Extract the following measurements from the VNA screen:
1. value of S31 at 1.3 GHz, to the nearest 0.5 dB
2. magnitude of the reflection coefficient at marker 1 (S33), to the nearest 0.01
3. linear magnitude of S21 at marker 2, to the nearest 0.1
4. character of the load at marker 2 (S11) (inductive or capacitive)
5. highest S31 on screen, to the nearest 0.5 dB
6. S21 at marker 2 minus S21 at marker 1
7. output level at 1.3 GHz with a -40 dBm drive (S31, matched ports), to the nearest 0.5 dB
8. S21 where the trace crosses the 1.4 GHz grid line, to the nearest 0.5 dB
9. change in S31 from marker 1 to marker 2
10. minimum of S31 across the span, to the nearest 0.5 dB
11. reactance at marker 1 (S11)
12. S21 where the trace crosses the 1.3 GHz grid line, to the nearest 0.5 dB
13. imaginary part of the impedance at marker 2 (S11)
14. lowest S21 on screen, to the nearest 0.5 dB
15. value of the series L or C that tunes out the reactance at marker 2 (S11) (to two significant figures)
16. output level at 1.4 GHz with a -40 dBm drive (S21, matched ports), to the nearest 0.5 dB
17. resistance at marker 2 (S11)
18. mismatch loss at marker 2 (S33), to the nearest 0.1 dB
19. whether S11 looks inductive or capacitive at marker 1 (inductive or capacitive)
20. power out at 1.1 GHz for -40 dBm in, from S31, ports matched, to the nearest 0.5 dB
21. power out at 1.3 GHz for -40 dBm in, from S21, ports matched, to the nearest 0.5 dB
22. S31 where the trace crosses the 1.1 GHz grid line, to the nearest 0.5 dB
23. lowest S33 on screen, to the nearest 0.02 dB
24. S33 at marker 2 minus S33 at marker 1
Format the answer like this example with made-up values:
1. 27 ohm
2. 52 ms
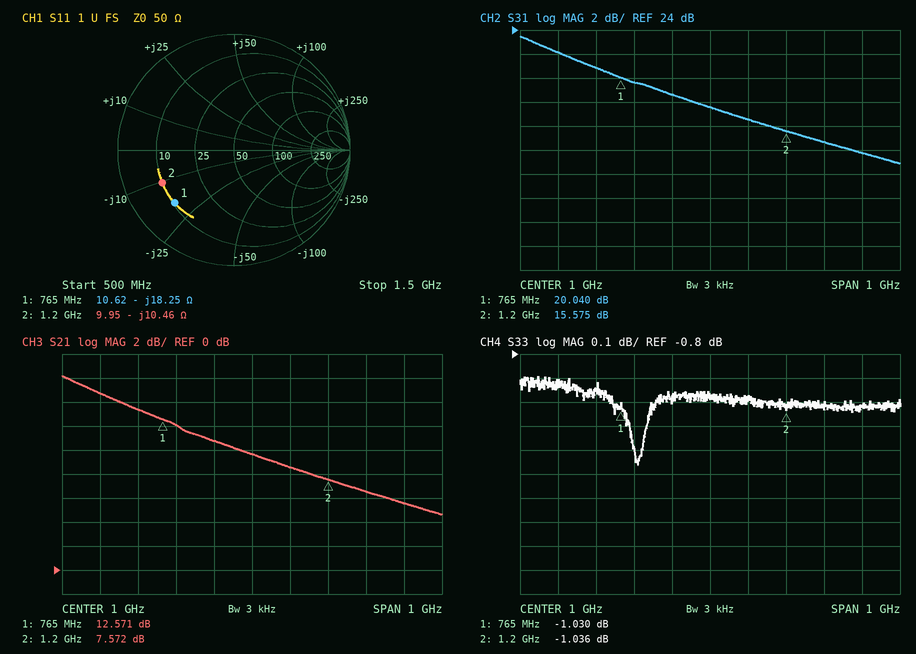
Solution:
1. 14.5 dB
2. 0.89
3. 2.4
4. capacitive
5. 23.5 dB
6. -4.999 dB
7. -25.5 dBm
8. 5.5 dB
9. -4.465 dB
10. 13.0 dB
11. -18.25 Ω
12. 6.5 dB
13. -10.46 Ω
14. 4.5 dB
15. 1.4 nH
16. -34.5 dBm
17. 9.95 Ω
18. 6.7 dB
19. capacitive
20. -23.5 dBm
21. -33.5 dBm
22. 16.5 dB
23. -1.26 dB
24. -0.006 dB
